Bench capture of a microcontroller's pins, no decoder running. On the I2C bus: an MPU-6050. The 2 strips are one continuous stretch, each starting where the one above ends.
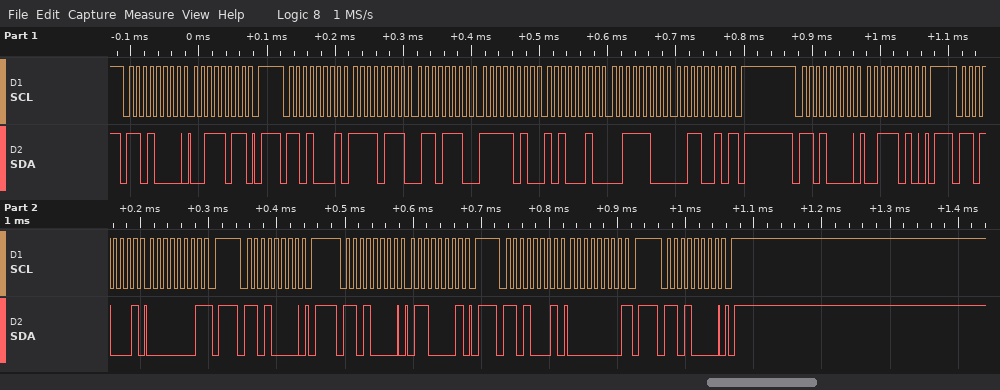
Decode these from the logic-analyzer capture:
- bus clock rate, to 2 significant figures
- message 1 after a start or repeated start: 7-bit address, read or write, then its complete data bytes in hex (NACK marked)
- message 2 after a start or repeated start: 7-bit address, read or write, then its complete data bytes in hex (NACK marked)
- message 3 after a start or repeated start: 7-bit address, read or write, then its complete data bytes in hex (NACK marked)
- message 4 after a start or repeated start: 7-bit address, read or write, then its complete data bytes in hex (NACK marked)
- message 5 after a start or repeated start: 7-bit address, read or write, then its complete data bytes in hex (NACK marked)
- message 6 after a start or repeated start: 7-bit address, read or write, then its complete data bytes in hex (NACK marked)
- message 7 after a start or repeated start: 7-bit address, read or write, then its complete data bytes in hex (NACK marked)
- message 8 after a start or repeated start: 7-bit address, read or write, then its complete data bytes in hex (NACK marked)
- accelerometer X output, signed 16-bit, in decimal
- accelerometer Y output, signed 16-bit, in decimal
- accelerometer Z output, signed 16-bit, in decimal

100 kHz
0x68 write: 3B
0x68 read: F7 6E FA A2 3C 32 NACK
0x68 write: 3A
0x68 read: 01 NACK
0x68 write
0x68 write: 61
0x68 read: 00 NACK
0x68 write
-2194
-1374
15410
